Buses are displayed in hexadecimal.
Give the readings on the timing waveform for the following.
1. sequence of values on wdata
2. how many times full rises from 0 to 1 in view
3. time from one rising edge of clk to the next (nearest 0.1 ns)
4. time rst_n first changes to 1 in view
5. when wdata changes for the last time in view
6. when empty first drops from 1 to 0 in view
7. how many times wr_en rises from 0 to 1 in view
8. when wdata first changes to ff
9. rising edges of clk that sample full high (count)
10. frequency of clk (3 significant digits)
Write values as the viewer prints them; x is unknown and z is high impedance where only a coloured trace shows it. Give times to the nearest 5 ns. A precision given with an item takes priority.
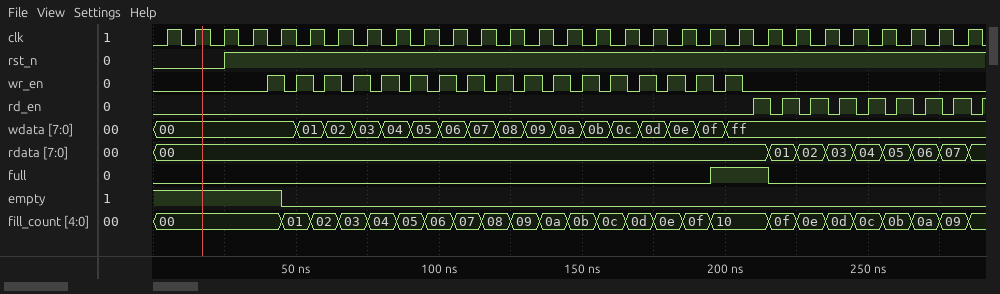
00, 01, 02, 03, 04, 05, 06, 07, 08, 09, 0a, 0b, 0c, 0d, 0e, 0f, ff
1
10 ns
25 ns
200 ns
45 ns
17
200 ns
2
100 MHz
